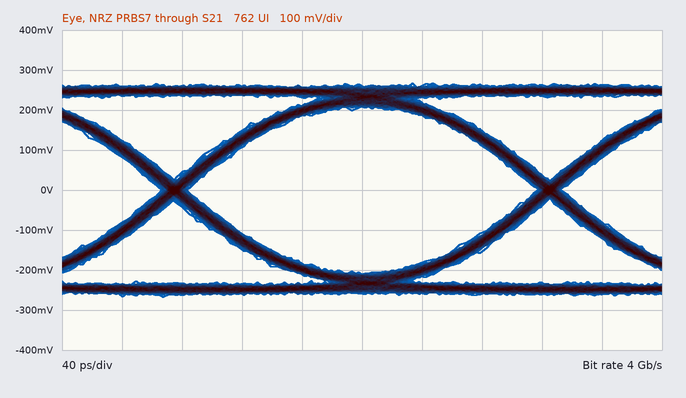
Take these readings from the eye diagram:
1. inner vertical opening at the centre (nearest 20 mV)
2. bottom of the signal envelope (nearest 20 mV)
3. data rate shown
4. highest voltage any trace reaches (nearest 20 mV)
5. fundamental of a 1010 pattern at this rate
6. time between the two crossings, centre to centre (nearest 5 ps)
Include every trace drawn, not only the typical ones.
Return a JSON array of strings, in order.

["420 mV", "-260 mV", "4 Gb/s", "260 mV", "2 GHz", "250 ps"]
